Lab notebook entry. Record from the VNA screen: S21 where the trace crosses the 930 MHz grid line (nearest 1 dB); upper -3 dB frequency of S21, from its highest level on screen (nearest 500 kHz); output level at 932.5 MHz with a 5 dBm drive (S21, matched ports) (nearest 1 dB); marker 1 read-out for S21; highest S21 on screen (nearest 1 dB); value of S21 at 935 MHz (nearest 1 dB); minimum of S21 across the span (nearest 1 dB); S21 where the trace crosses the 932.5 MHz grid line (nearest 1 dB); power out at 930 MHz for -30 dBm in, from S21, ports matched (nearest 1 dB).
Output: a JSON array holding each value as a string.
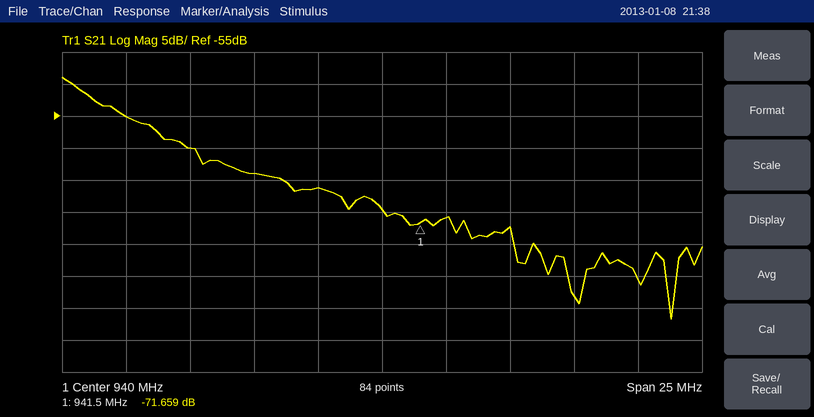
["-55 dB", "928.5 MHz", "-55 dBm", "-71.659 dB", "-49 dB", "-64 dB", "-87 dB", "-60 dB", "-85 dBm"]
